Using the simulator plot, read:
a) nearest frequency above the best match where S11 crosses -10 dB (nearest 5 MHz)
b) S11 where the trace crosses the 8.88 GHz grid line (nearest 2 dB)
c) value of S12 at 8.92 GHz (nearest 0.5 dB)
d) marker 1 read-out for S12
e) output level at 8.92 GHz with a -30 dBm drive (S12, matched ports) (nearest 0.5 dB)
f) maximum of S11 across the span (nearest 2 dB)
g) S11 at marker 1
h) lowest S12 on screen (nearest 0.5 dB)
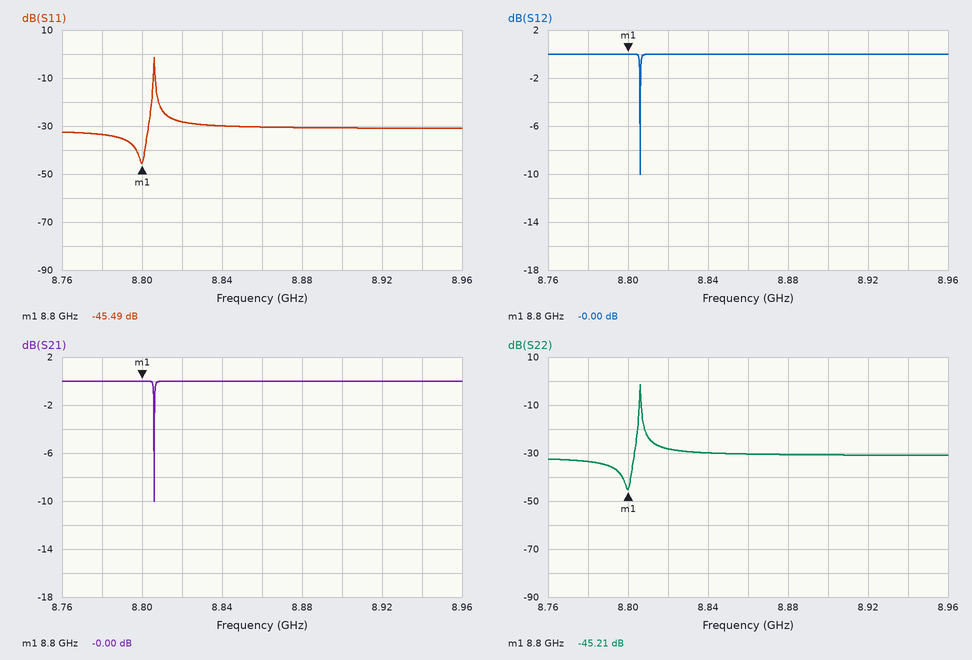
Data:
8.805 GHz
-30 dB
0.0 dB
-0.00 dB
-30.0 dBm
-2 dB
-45.49 dB
-10.0 dB
